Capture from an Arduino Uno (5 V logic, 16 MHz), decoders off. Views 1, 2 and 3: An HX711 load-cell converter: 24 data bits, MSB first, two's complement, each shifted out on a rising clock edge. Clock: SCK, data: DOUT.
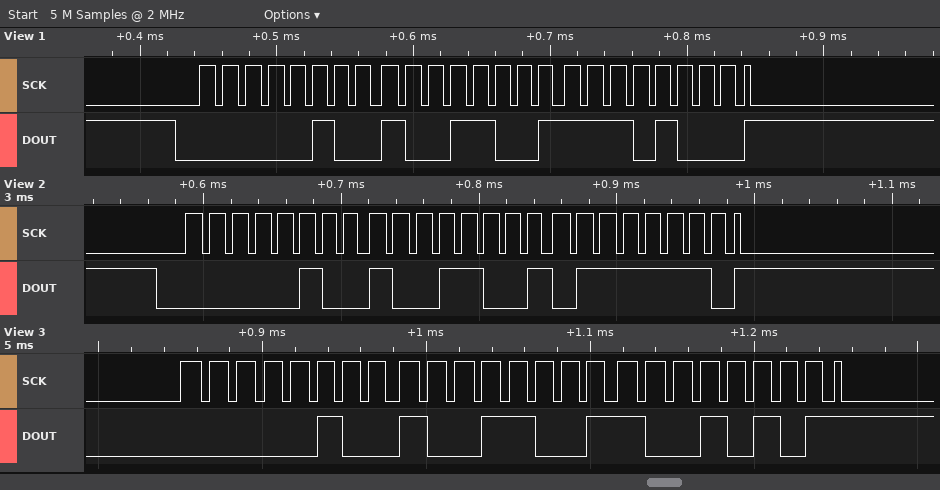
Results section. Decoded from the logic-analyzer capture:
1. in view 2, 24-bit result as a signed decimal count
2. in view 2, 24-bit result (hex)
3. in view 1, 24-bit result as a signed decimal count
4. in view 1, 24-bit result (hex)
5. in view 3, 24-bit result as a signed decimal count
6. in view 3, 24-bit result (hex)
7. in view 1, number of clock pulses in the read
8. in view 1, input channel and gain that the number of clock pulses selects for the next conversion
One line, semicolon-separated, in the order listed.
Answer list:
301438; 0x04997E; 301544; 0x0499E8; 301461; 0x049995; 25; channel A, gain 128
